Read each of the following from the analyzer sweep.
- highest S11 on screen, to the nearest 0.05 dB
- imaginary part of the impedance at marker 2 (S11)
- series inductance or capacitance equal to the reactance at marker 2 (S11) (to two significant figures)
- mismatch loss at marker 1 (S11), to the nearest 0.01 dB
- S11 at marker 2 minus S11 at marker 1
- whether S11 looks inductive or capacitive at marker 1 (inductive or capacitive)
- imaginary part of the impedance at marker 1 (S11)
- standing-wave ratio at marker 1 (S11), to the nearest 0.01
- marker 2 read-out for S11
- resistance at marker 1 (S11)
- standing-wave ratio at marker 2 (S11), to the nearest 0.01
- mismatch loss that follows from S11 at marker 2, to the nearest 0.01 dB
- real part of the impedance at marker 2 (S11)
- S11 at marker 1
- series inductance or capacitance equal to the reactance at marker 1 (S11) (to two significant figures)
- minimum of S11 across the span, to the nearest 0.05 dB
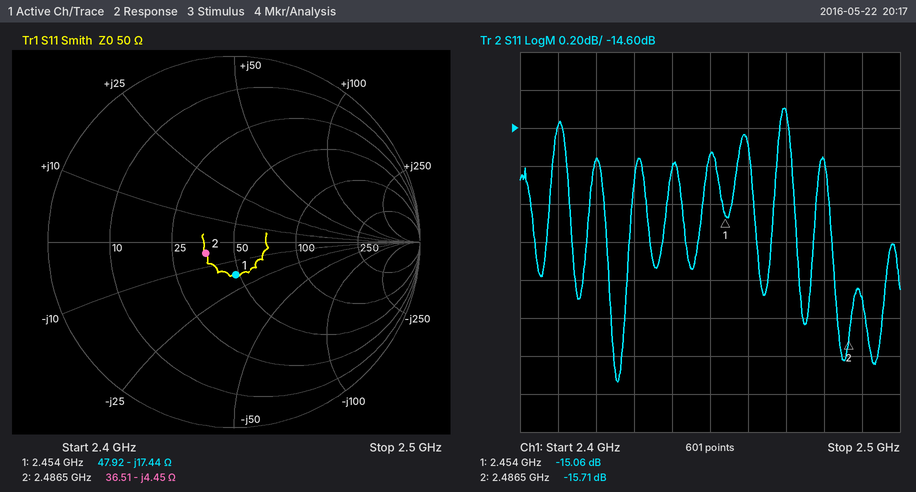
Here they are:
-14.50 dB
-4.45 Ω
14 pF
0.14 dB
-0.65 dB
capacitive
-17.44 Ω
1.43
-15.71 dB
47.92 Ω
1.39
0.12 dB
36.51 Ω
-15.06 dB
3.7 pF
-15.95 dB
